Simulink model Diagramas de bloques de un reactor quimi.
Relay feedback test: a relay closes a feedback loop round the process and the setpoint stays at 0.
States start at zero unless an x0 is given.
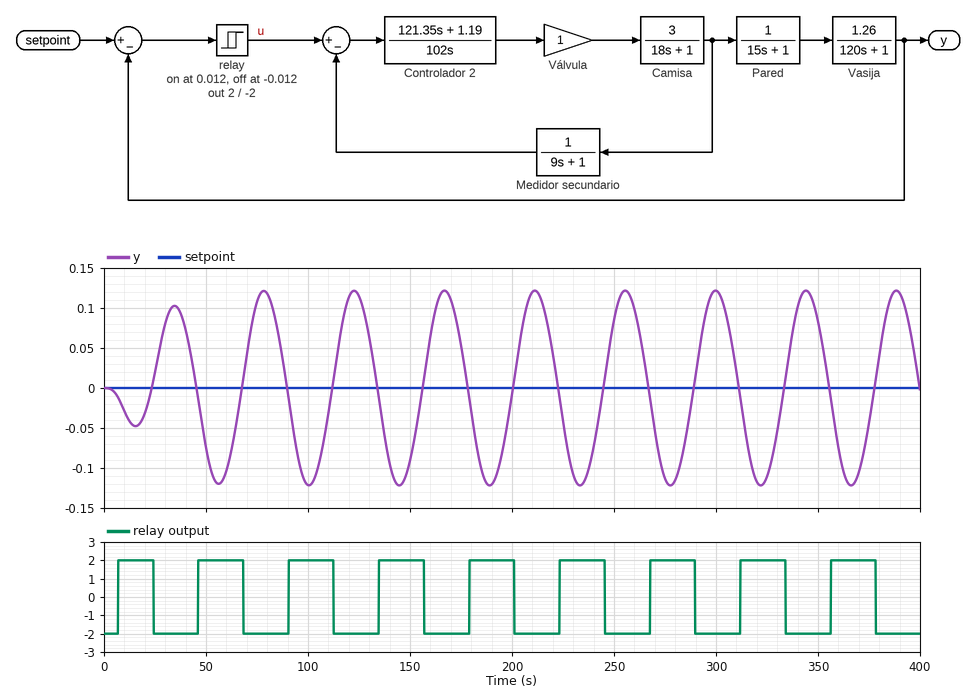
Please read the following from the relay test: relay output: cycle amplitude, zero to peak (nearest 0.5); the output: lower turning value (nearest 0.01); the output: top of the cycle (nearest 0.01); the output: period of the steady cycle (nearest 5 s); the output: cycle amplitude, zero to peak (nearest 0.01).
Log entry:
2.0
-0.12
0.12
45 s
0.12
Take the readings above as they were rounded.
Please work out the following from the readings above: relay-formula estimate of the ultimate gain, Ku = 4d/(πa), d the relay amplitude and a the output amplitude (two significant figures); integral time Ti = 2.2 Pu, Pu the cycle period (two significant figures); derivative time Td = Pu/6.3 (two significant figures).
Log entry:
21
99 s
7.1 s
